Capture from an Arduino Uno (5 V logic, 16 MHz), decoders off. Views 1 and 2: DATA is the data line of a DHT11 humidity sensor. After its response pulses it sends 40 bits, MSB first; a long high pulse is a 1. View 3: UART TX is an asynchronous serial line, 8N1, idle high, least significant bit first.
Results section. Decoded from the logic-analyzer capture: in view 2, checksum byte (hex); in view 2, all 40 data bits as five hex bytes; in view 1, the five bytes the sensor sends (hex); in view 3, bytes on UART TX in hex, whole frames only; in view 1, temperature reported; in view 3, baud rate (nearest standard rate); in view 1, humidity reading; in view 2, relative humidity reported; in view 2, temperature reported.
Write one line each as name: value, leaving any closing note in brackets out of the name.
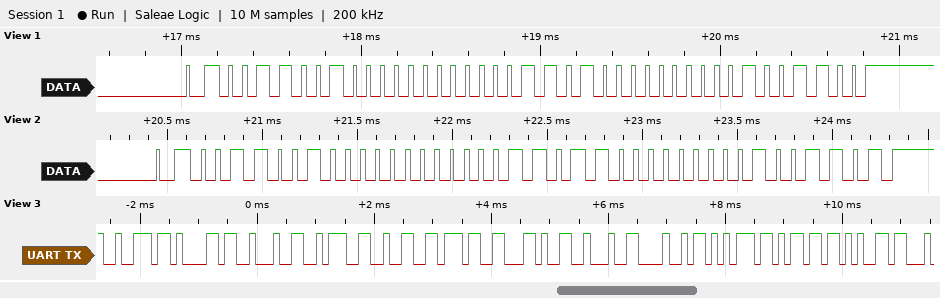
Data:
in view 2, checksum byte: 0x4D
in view 2, all 40 data bits as five hex bytes: 32 00 1B 00 4D
in view 1, the five bytes the sensor sends: 32 00 1A 00 4C
in view 3, bytes on UART TX in hex, whole frames only: 0x72 0x61 0x22 0x3A 0x32 0x37 0x2C 0x22 0x48 0x75 0x6D 0x65
in view 1, temperature reported: 26.0 °C
in view 3, baud rate: 9600 baud
in view 1, humidity reading: 50 %
in view 2, relative humidity reported: 50 %
in view 2, temperature reported: 27.0 °C
